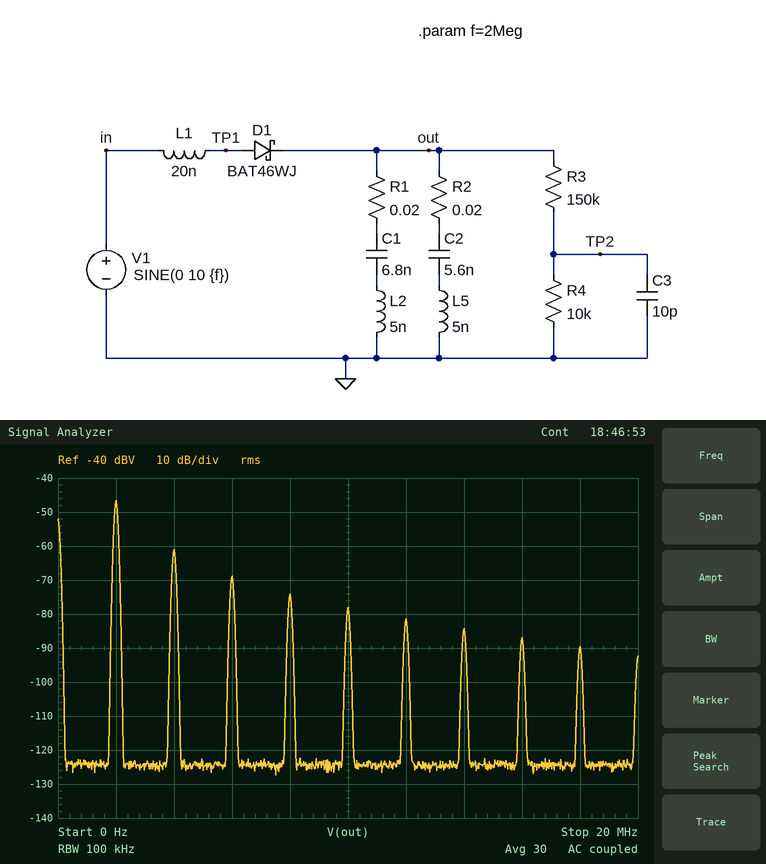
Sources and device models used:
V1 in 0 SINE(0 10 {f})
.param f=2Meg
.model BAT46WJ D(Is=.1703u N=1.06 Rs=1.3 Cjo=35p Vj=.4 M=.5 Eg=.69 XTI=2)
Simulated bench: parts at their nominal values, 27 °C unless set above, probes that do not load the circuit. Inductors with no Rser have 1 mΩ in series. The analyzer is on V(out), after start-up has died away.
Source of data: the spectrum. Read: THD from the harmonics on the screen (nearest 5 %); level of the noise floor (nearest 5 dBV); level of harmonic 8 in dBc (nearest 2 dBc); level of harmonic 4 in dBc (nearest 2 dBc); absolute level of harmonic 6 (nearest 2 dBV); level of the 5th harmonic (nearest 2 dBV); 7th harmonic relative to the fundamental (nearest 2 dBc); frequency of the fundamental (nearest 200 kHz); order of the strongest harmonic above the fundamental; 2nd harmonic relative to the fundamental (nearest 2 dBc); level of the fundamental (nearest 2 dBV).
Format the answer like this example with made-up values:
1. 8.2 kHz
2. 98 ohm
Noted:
1. 20 %
2. -125 dBV
3. -40 dBc
4. -28 dBc
5. -82 dBV
6. -78 dBV
7. -38 dBc
8. 2.0 MHz
9. 2
10. -14 dBc
11. -46 dBV
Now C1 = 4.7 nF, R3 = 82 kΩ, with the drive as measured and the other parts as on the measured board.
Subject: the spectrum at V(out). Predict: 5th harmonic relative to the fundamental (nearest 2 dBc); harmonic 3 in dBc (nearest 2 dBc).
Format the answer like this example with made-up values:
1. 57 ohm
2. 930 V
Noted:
1. -28 dBc
2. -20 dBc
